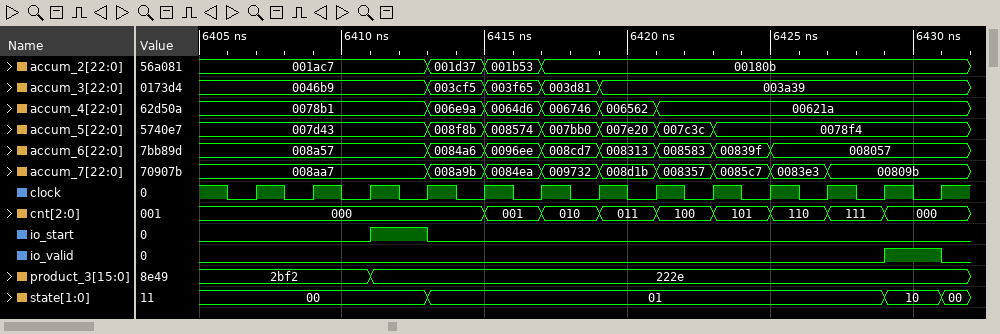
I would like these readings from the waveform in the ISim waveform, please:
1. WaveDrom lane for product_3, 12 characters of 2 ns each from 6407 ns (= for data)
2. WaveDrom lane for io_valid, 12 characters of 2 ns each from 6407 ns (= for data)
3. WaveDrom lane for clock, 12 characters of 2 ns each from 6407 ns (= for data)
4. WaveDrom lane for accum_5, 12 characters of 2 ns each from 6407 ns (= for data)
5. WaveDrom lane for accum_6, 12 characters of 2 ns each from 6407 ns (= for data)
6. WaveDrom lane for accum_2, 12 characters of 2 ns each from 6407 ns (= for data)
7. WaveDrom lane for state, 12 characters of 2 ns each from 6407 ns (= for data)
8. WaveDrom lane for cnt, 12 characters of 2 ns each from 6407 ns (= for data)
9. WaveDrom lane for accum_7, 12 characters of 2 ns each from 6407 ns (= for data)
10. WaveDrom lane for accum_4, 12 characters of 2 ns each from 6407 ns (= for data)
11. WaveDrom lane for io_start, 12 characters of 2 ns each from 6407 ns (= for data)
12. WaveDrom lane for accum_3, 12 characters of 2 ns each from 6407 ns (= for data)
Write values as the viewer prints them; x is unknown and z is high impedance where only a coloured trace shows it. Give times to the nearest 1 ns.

{name: 'product_3', wave: '=.=.........', data: '2bf2 222e'}
{name: 'io_valid', wave: '0..........1'}
{name: 'clock', wave: 'p...........'}
{name: 'accum_5', wave: '=..======...', data: '007d43 008f8b 008574 007bb0 007e20 007c3c 0078f4'}
{name: 'accum_6', wave: '=..=======..', data: '008a57 0084a6 0096ee 008cd7 008313 008583 00839f 008057'}
{name: 'accum_2', wave: '=..===......', data: '001ac7 001d37 001b53 00180b'}
{name: 'state', wave: '=..=.......=', data: '00 01 10'}
{name: 'cnt', wave: '=...========', data: '000 001 010 011 100 101 110 111 000'}
{name: 'accum_7', wave: '=..========.', data: '008aa7 008a9b 0084ea 009732 008d1b 008357 0085c7 0083e3 00809b'}
{name: 'accum_4', wave: '=..=====....', data: '0078b1 006e9a 0064d6 006746 006562 00621a'}
{name: 'io_start', wave: '0.10........'}
{name: 'accum_3', wave: '=..====.....', data: '0046b9 003cf5 003f65 003d81 003a39'}
